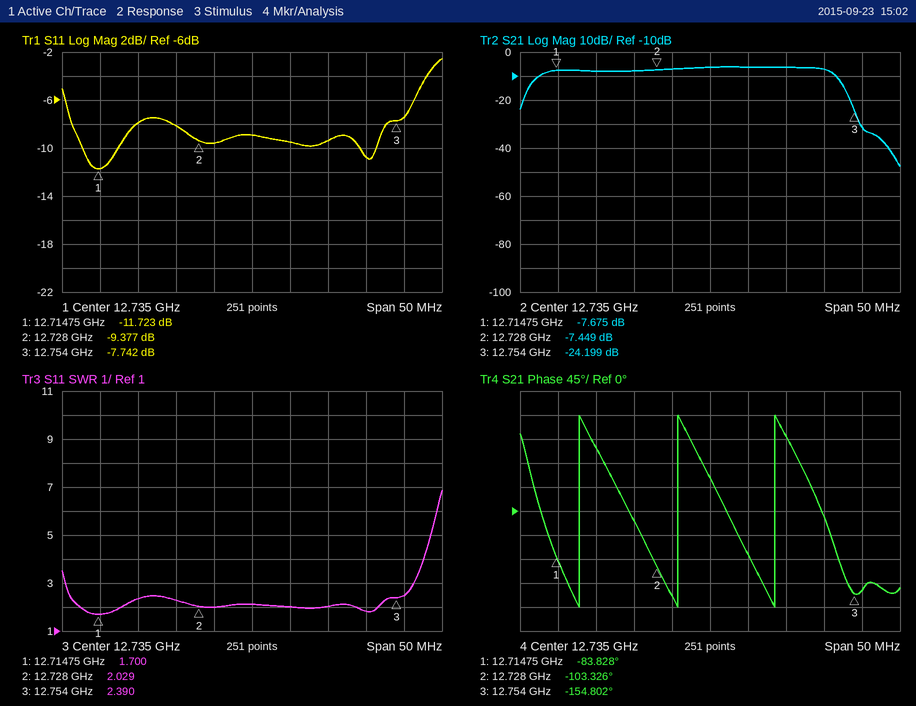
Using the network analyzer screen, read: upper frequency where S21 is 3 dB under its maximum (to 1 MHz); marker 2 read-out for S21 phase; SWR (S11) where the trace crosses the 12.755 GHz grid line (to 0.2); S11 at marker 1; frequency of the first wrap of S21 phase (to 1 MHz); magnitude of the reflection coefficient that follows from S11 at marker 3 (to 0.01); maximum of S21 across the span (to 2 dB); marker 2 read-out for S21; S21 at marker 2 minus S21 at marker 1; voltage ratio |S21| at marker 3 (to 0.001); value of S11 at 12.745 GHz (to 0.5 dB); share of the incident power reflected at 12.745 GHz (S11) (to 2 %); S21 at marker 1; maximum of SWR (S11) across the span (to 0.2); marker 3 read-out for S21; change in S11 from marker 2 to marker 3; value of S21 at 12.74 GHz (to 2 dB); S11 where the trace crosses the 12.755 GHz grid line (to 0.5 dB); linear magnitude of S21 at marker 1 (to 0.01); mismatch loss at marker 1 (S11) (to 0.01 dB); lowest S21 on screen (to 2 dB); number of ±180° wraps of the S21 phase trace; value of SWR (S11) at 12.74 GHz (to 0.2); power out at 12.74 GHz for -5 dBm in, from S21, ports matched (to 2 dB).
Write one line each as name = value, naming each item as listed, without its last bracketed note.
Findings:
upper frequency where S21 is 3 dB under its maximum = 12.751 GHz
marker 2 read-out for S21 phase = -103.326°
SWR (S11) where the trace crosses the 12.755 GHz grid line = 2.4
S11 at marker 1 = -11.723 dB
frequency of the first wrap of S21 phase = 12.718 GHz
magnitude of the reflection coefficient that follows from S11 at marker 3 = 0.41
maximum of S21 across the span = -6 dB
marker 2 read-out for S21 = -7.449 dB
S21 at marker 2 minus S21 at marker 1 = 0.226 dB
voltage ratio |S21| at marker 3 = 0.062
value of S11 at 12.745 GHz = -9.5 dB
share of the incident power reflected at 12.745 GHz (S11) = 12 %
S21 at marker 1 = -7.675 dB
maximum of SWR (S11) across the span = 6.8
marker 3 read-out for S21 = -24.199 dB
change in S11 from marker 2 to marker 3 = 1.635 dB
value of S21 at 12.74 GHz = -6 dB
S11 where the trace crosses the 12.755 GHz grid line = -7.5 dB
linear magnitude of S21 at marker 1 = 0.41
mismatch loss at marker 1 (S11) = 0.30 dB
lowest S21 on screen = -48 dB
number of ±180° wraps of the S21 phase trace = 3
value of SWR (S11) at 12.74 GHz = 2.0
power out at 12.74 GHz for -5 dBm in, from S21, ports matched = -12 dBm
